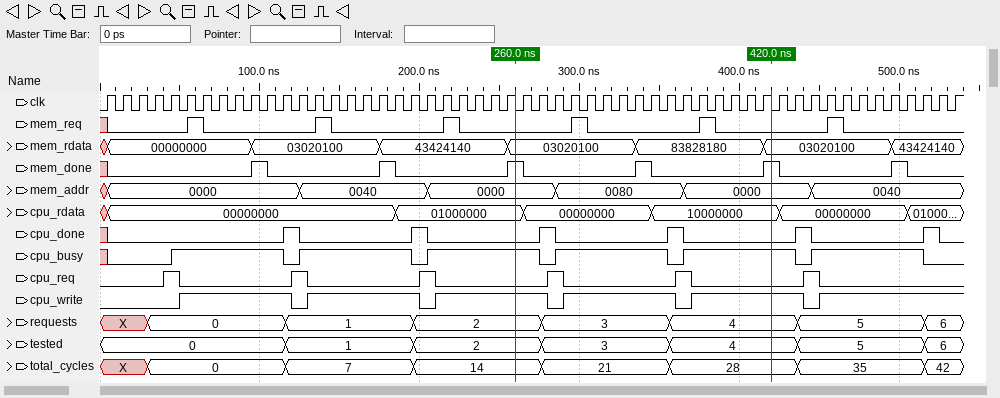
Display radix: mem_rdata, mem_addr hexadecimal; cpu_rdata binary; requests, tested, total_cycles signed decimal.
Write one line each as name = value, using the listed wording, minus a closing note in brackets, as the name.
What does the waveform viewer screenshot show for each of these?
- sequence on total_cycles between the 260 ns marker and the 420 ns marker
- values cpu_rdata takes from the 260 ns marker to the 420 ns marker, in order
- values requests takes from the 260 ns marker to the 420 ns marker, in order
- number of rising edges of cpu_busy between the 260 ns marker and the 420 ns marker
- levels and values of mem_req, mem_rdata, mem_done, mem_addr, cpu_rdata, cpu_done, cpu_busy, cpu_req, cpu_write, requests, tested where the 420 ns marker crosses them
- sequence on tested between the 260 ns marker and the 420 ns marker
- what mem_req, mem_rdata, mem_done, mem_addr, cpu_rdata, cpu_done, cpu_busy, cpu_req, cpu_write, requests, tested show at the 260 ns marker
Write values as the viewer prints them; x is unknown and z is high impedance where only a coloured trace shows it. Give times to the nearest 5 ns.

sequence on total_cycles between the 260 ns marker and the 420 ns marker = 14, 21, 28
values cpu_rdata takes from the 260 ns marker to the 420 ns marker, in order = 01000000, 00000000, 10000000
values requests takes from the 260 ns marker to the 420 ns marker, in order = 2, 3, 4
number of rising edges of cpu_busy between the 260 ns marker and the 420 ns marker = 2
levels and values of mem_req, mem_rdata, mem_done, mem_addr, cpu_rdata, cpu_done, cpu_busy, cpu_req, cpu_write, requests, tested where the 420 ns marker crosses them = mem_req=0, mem_rdata=03020100, mem_done=1, mem_addr=0000, cpu_rdata=10000000, cpu_done=0, cpu_busy=1, cpu_req=0, cpu_write=1, requests=4, tested=4
sequence on tested between the 260 ns marker and the 420 ns marker = 2, 3, 4
what mem_req, mem_rdata, mem_done, mem_addr, cpu_rdata, cpu_done, cpu_busy, cpu_req, cpu_write, requests, tested show at the 260 ns marker = mem_req=0, mem_rdata=03020100, mem_done=1, mem_addr=0000, cpu_rdata=01000000, cpu_done=0, cpu_busy=1, cpu_req=0, cpu_write=1, requests=2, tested=2
